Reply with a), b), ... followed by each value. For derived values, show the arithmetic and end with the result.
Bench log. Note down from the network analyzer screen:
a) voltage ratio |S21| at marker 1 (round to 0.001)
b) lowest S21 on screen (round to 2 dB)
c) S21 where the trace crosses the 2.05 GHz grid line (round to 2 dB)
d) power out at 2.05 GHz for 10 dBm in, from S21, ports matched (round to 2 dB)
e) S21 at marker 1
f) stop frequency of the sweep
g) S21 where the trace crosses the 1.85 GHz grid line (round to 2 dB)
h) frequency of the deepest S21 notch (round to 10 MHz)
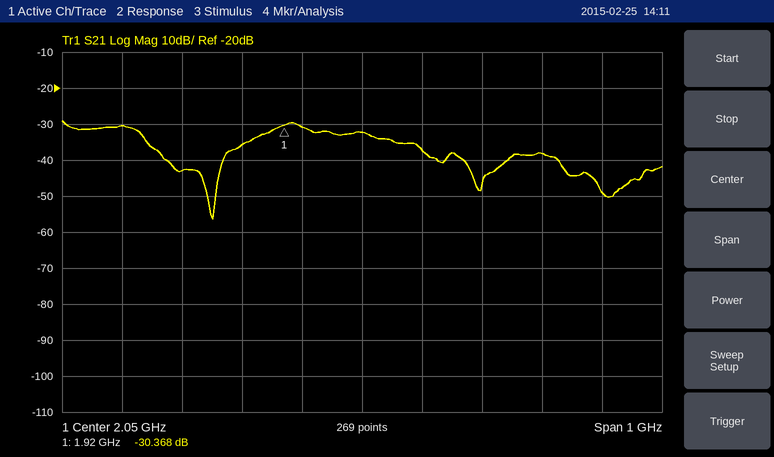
a) 10^(-30.368/20) ≈ 0.030
b) -56 dB
c) -32 dB
d) 10 dBm + (-32 dB) = -22 dBm
e) -30.368 dB
f) 2.55 GHz
g) -36 dB
h) 1.80 GHz
